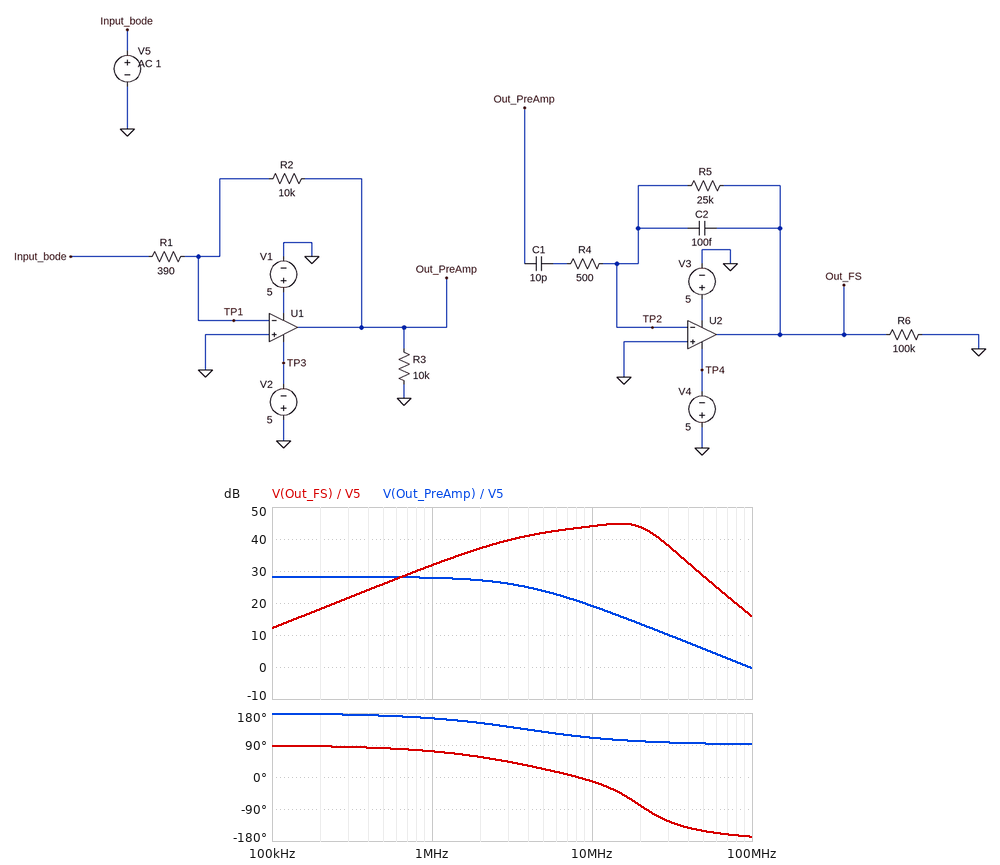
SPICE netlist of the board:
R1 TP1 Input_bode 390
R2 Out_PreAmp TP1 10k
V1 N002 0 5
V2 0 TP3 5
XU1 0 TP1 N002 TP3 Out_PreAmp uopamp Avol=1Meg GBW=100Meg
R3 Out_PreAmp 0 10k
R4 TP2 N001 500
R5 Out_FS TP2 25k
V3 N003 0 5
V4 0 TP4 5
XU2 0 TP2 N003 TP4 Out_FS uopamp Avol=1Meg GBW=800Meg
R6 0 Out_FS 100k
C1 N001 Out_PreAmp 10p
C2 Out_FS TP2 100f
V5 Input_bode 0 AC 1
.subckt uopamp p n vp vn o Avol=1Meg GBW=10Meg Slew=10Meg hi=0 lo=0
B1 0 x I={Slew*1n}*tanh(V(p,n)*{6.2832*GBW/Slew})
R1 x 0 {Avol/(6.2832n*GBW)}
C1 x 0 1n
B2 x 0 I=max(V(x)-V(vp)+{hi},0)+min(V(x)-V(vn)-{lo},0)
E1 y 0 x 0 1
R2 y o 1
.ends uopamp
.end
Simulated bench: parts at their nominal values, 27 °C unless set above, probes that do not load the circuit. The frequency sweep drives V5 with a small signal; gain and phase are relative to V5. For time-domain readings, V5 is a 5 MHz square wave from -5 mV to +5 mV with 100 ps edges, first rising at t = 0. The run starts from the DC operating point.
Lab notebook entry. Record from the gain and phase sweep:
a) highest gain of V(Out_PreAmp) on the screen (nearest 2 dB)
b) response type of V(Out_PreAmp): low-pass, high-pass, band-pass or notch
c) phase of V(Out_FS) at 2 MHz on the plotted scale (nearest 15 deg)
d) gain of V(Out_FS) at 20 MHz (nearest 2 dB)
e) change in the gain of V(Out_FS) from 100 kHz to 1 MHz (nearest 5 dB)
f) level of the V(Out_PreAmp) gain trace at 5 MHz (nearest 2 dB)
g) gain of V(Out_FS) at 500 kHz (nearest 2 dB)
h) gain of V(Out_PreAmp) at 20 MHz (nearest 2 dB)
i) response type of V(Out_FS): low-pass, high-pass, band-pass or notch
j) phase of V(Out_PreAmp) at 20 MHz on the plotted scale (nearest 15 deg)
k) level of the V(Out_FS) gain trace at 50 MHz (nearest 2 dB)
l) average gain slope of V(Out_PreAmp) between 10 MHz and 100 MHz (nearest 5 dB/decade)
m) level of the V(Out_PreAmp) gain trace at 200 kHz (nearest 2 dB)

28 dB
low-pass
60 deg
44 dB
20 dB
24 dB
26 dB
14 dB
band-pass
105 deg
28 dB
-20 dB/decade
28 dB
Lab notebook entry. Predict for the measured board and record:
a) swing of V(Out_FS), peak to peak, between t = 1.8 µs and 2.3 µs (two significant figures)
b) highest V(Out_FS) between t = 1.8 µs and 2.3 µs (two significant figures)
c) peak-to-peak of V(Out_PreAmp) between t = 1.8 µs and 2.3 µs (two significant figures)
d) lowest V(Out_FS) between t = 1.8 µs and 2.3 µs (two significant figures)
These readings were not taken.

1.0 V
500 mV
210 mV
-500 mV
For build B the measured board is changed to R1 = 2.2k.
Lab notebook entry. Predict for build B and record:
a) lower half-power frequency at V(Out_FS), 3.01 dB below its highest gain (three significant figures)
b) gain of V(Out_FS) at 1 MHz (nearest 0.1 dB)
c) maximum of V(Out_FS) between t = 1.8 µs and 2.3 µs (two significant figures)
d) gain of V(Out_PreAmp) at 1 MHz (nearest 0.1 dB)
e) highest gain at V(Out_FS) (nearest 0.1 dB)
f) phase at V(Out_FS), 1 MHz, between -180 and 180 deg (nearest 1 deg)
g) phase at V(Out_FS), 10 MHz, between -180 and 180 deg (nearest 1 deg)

10.4 MHz
17.1 dB
490 mV
13.1 dB
40.2 dB
84 deg
28 deg
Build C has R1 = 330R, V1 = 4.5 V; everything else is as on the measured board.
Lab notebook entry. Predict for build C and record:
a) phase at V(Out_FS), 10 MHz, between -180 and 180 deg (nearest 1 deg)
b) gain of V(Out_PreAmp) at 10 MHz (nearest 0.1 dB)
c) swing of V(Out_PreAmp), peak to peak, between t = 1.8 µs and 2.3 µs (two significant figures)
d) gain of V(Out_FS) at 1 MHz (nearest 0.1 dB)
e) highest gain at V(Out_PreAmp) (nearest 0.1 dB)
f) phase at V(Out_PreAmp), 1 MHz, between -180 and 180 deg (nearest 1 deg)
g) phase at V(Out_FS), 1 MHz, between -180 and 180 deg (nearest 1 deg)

-15 deg
19.3 dB
230 mV
33.2 dB
29.6 dB
163 deg
70 deg
